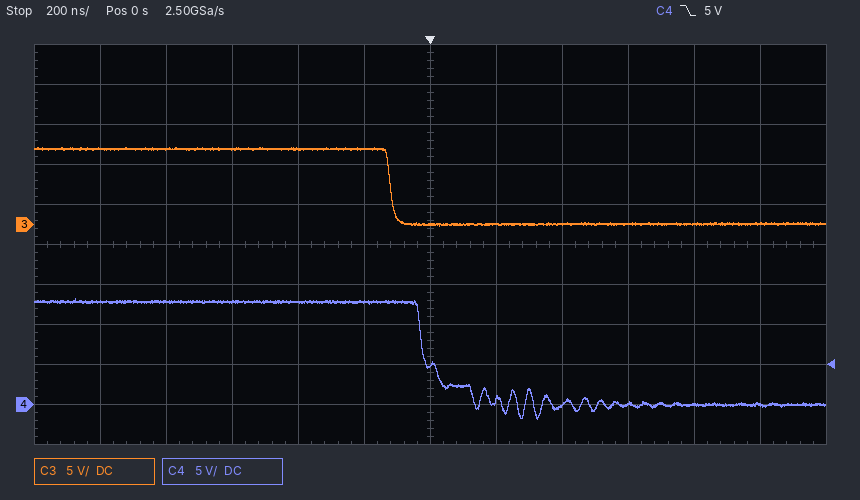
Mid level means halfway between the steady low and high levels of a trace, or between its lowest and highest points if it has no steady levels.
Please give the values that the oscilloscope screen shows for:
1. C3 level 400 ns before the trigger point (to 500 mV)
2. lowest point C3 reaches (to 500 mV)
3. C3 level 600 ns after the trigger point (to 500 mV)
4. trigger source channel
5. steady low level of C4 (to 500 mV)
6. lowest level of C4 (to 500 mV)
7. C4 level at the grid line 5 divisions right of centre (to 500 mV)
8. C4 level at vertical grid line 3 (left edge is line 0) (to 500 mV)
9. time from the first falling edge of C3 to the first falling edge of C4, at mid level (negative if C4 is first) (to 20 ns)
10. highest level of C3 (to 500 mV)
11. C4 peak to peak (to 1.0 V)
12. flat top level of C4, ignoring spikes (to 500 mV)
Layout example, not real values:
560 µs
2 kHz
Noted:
9.5 V
0.0 V
0.0 V
C4
0.0 V
-2.0 V
0.0 V
13.0 V
+100 ns
9.5 V
15.0 V
13.0 V
